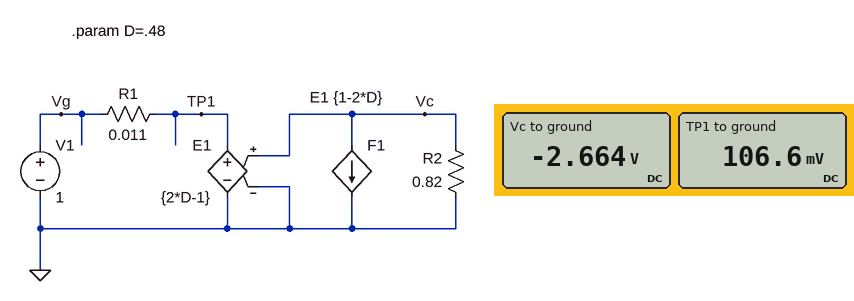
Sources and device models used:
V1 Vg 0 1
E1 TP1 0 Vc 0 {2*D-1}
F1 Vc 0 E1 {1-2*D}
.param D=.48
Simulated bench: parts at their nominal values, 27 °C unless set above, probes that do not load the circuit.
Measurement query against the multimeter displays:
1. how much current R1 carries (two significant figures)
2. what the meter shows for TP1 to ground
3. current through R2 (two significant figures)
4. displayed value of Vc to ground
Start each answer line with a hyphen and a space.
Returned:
- 81 A
- 106.6 mV
- 3.2 A
- -2.664 V
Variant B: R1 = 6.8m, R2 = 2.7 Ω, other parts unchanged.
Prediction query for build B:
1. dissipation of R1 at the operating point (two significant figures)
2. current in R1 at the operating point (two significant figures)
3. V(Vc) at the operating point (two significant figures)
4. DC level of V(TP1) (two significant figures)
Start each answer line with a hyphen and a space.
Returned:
- 55 W
- 90 A
- -9.7 V
- 390 mV
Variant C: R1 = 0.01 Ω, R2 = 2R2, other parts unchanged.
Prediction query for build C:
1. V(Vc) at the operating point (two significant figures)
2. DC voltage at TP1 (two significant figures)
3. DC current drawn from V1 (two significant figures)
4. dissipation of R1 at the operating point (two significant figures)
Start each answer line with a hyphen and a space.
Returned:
- -6.5 V
- 260 mV
- 74 A
- 55 W
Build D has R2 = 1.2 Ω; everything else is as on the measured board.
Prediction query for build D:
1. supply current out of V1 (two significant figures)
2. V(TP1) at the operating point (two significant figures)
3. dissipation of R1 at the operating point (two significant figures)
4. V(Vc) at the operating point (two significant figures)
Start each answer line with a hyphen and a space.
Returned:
- 77 A
- 150 mV
- 66 W
- -3.7 V
